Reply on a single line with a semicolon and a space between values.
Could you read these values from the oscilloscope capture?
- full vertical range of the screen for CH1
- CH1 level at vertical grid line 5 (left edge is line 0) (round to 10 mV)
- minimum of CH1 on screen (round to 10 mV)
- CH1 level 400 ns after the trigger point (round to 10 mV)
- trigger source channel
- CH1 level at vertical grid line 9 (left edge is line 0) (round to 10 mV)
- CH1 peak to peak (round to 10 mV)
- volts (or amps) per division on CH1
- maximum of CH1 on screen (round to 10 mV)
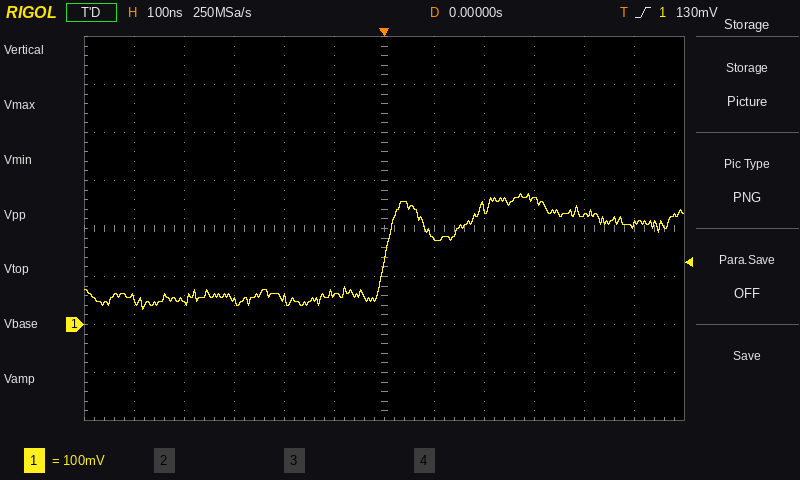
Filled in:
800 mV; 60 mV; 30 mV; 230 mV; CH1; 260 mV; 240 mV; 100 mV; 270 mV
